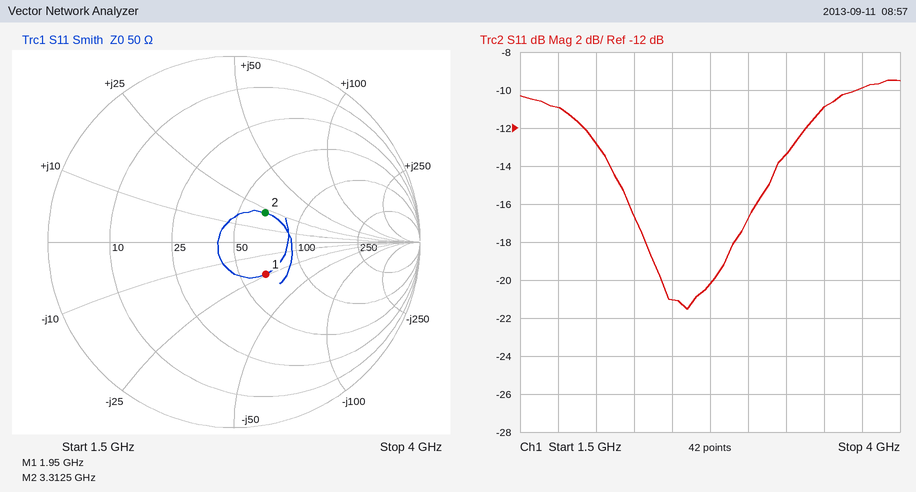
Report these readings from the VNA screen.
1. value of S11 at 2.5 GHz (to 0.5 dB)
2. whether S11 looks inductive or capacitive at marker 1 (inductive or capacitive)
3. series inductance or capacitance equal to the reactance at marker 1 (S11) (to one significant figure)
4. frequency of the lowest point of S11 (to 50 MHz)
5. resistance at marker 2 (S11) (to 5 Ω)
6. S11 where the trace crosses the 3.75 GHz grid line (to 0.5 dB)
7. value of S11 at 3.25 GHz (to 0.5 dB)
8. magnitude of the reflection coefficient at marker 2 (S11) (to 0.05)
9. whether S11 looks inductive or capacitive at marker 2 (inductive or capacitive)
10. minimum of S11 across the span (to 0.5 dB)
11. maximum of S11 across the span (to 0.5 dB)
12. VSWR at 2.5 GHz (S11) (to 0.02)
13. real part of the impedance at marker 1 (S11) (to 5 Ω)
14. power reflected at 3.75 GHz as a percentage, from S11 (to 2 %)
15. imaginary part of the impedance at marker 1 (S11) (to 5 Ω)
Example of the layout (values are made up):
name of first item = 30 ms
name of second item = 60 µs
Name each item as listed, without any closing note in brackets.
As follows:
value of S11 at 2.5 GHz = -21.0 dB
whether S11 looks inductive or capacitive at marker 1 = capacitive
series inductance or capacitance equal to the reactance at marker 1 (S11) = 3 pF
frequency of the lowest point of S11 = 2.60 GHz
resistance at marker 2 (S11) = 65 Ω
S11 where the trace crosses the 3.75 GHz grid line = -10.0 dB
value of S11 at 3.25 GHz = -13.5 dB
magnitude of the reflection coefficient at marker 2 (S11) = 0.25
whether S11 looks inductive or capacitive at marker 2 = inductive
minimum of S11 across the span = -21.5 dB
maximum of S11 across the span = -9.5 dB
VSWR at 2.5 GHz (S11) = 1.20
real part of the impedance at marker 1 (S11) = 65 Ω
power reflected at 3.75 GHz as a percentage, from S11 = 10 %
imaginary part of the impedance at marker 1 (S11) = -25 Ω
